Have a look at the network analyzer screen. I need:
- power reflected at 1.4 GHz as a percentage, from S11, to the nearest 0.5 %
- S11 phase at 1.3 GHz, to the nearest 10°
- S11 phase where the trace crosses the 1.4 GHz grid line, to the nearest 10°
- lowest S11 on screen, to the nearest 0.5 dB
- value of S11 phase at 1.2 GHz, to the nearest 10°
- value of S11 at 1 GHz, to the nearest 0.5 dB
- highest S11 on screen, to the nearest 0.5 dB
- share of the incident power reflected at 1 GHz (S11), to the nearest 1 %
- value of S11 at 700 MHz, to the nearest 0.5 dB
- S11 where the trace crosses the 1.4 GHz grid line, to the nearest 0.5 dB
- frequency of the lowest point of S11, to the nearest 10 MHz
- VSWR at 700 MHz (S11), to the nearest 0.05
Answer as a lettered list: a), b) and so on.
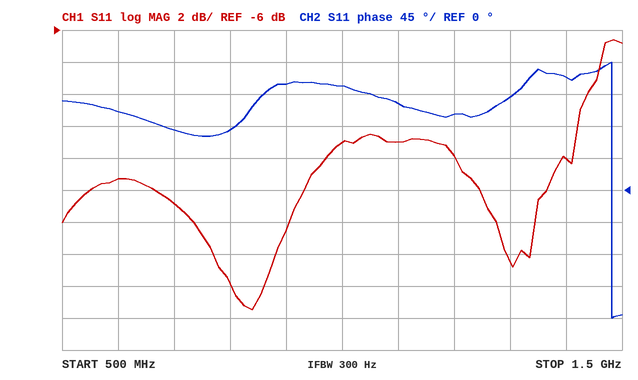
a) 4.0 %
b) 130°
c) 160°
d) -23.5 dB
e) 110°
f) -13.0 dB
g) -6.5 dB
h) 5 %
i) -17.0 dB
j) -14.0 dB
k) 840 MHz
l) 1.35
